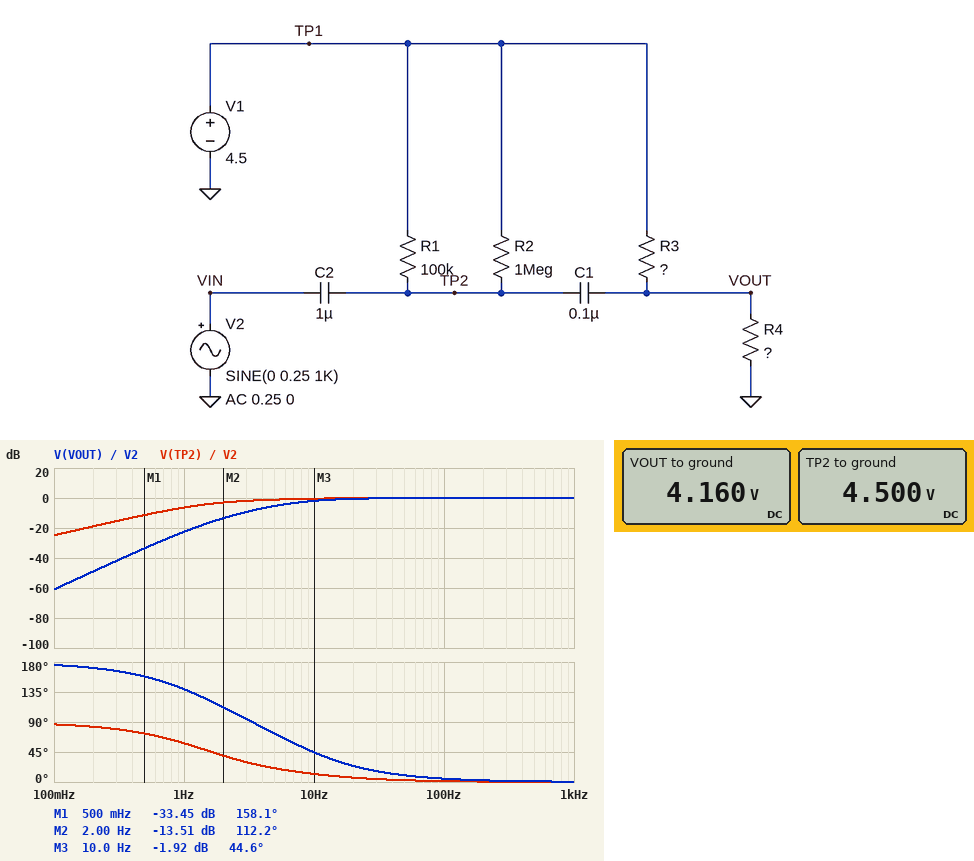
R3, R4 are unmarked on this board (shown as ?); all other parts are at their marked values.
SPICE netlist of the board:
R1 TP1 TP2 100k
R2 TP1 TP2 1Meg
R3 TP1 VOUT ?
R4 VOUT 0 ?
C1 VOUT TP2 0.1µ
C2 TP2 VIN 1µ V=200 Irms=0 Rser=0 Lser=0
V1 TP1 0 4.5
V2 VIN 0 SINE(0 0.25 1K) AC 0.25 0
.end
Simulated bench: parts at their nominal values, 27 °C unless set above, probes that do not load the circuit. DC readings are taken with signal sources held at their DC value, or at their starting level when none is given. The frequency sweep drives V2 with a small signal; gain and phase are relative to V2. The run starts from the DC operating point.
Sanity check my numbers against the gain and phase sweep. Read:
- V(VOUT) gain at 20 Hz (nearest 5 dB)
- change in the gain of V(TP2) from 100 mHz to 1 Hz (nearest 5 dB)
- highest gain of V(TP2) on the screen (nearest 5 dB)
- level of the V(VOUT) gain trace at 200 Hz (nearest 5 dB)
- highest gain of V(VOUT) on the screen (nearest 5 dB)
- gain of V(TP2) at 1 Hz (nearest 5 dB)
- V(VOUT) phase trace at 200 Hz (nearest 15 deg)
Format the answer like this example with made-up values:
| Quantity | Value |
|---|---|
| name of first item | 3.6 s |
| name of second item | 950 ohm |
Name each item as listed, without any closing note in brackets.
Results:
| Quantity | Value |
|---|---|
| V(VOUT) gain at 20 Hz | 0 dB |
| change in the gain of V(TP2) from 100 mHz to 1 Hz | 20 dB |
| highest gain of V(TP2) on the screen | 0 dB |
| level of the V(VOUT) gain trace at 200 Hz | 0 dB |
| highest gain of V(VOUT) on the screen | 0 dB |
| gain of V(TP2) at 1 Hz | -5 dB |
| V(VOUT) phase trace at 200 Hz | 0 deg |
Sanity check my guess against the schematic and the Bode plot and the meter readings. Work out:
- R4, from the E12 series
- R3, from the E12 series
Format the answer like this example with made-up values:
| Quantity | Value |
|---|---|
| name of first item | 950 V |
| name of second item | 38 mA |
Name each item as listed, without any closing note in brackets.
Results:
| Quantity | Value |
|---|---|
| R4, from the E12 series | 3.3 MΩ |
| R3, from the E12 series | 270 kΩ |
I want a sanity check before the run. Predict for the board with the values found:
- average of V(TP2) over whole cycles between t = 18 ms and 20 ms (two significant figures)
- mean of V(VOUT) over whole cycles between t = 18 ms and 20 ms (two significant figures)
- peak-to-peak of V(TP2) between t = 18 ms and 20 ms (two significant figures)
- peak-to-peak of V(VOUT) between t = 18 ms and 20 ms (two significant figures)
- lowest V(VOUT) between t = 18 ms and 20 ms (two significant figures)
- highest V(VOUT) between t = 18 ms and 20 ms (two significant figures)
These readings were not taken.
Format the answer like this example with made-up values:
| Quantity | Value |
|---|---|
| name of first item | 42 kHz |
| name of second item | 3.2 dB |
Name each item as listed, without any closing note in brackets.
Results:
| Quantity | Value |
|---|---|
| average of V(TP2) over whole cycles between t = 18 ms and 20 ms | 4.5 V |
| mean of V(VOUT) over whole cycles between t = 18 ms and 20 ms | 4.2 V |
| peak-to-peak of V(TP2) between t = 18 ms and 20 ms | 500 mV |
| peak-to-peak of V(VOUT) between t = 18 ms and 20 ms | 500 mV |
| lowest V(VOUT) between t = 18 ms and 20 ms | 3.9 V |
| highest V(VOUT) between t = 18 ms and 20 ms | 4.4 V |
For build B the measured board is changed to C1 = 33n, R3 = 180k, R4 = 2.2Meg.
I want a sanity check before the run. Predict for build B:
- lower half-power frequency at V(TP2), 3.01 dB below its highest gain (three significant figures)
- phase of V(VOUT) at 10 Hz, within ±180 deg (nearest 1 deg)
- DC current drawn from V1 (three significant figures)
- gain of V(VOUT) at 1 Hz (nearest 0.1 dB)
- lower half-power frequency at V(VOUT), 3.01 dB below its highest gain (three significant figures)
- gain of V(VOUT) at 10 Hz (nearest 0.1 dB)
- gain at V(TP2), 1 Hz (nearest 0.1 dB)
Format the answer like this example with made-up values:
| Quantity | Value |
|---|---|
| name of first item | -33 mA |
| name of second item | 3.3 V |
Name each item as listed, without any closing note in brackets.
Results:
| Quantity | Value |
|---|---|
| lower half-power frequency at V(TP2), 3.01 dB below its highest gain | 1.82 Hz |
| phase of V(VOUT) at 10 Hz, within ±180 deg | 81 deg |
| DC current drawn from V1 | 1.89 µA |
| gain of V(VOUT) at 1 Hz | -35.4 dB |
| lower half-power frequency at V(VOUT), 3.01 dB below its highest gain | 30.1 Hz |
| gain of V(VOUT) at 10 Hz | -10.1 dB |
| gain at V(TP2), 1 Hz | -6.2 dB |
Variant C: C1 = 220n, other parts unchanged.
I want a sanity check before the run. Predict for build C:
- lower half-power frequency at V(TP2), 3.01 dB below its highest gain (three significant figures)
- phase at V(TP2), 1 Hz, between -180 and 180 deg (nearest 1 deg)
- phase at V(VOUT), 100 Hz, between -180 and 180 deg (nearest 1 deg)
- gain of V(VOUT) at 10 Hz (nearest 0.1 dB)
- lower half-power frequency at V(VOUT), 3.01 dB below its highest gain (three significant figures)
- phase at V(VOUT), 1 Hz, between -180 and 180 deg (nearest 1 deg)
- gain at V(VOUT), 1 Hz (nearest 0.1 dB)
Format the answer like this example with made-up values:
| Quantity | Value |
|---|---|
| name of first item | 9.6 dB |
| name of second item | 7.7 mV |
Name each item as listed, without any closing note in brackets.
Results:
| Quantity | Value |
|---|---|
| lower half-power frequency at V(TP2), 3.01 dB below its highest gain | 2.37 Hz |
| phase at V(TP2), 1 Hz, between -180 and 180 deg | 57 deg |
| phase at V(VOUT), 100 Hz, between -180 and 180 deg | 3 deg |
| gain of V(VOUT) at 10 Hz | -0.7 dB |
| lower half-power frequency at V(VOUT), 3.01 dB below its highest gain | 4.38 Hz |
| phase at V(VOUT), 1 Hz, between -180 and 180 deg | 128 deg |
| gain at V(VOUT), 1 Hz | -16.5 dB |
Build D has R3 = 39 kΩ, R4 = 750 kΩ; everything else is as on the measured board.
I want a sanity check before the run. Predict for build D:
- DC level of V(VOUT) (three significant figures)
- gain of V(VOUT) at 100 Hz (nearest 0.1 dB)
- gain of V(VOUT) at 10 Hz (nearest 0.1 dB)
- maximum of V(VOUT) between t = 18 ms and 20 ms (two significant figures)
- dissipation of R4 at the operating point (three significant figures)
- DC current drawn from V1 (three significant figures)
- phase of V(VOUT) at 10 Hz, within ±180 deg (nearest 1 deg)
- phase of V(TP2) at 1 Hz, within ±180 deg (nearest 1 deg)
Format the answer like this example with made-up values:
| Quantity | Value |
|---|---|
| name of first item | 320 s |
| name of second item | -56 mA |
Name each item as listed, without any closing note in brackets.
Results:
| Quantity | Value |
|---|---|
| DC level of V(VOUT) | 4.28 V |
| gain of V(VOUT) at 100 Hz | -0.9 dB |
| gain of V(VOUT) at 10 Hz | -13.8 dB |
| maximum of V(VOUT) between t = 18 ms and 20 ms | 4.5 V |
| dissipation of R4 at the operating point | 24.4 µW |
| DC current drawn from V1 | 5.70 µA |
| phase of V(VOUT) at 10 Hz, within ±180 deg | 87 deg |
| phase of V(TP2) at 1 Hz, within ±180 deg | 58 deg |
